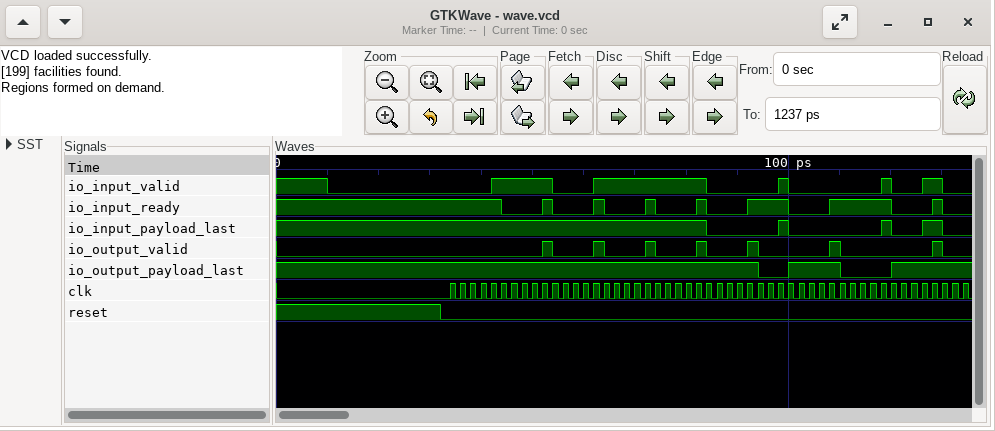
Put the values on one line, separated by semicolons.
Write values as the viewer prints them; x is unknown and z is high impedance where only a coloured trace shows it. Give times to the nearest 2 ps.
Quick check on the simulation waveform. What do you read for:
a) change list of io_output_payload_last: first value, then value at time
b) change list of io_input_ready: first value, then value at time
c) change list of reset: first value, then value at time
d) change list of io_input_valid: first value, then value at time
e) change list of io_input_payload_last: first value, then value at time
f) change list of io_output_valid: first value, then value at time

1, 0 at 94 ps, 1 at 100 ps, 0 at 110 ps, 1 at 120 ps; 1, 0 at 44 ps, 1 at 52 ps, 0 at 54 ps, 1 at 62 ps, 0 at 64 ps, 1 at 72 ps, 0 at 74 ps, 1 at 82 ps, 0 at 84 ps, 1 at 92 ps, 0 at 100 ps, 1 at 108 ps, 0 at 120 ps, 1 at 128 ps, 0 at 130 ps; 1, 0 at 32 ps; 1, 0 at 10 ps, 1 at 42 ps, 0 at 54 ps, 1 at 62 ps, 0 at 84 ps, 1 at 98 ps, 0 at 100 ps, 1 at 118 ps, 0 at 120 ps, 1 at 126 ps, 0 at 130 ps; 1, 0 at 84 ps, 1 at 98 ps, 0 at 100 ps, 1 at 118 ps, 0 at 120 ps, 1 at 126 ps, 0 at 130 ps; 0, 1 at 52 ps, 0 at 54 ps, 1 at 62 ps, 0 at 64 ps, 1 at 72 ps, 0 at 74 ps, 1 at 82 ps, 0 at 84 ps, 1 at 92 ps, 0 at 94 ps, 1 at 108 ps, 0 at 110 ps, 1 at 128 ps, 0 at 130 ps
